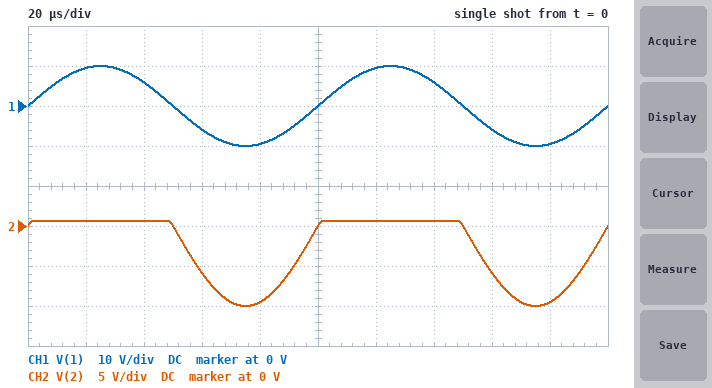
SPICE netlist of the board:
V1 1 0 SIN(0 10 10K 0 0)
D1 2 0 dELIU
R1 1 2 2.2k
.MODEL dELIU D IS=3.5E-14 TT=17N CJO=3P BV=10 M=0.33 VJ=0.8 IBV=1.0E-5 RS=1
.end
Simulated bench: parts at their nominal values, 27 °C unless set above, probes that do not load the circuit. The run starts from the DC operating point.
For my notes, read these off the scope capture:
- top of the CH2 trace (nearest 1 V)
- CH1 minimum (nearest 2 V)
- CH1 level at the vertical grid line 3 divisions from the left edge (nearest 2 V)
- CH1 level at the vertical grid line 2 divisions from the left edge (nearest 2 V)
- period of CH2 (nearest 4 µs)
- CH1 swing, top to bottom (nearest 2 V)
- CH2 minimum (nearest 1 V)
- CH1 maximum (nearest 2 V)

1 V
-10 V
-6 V
6 V
100 µs
20 V
-10 V
10 V
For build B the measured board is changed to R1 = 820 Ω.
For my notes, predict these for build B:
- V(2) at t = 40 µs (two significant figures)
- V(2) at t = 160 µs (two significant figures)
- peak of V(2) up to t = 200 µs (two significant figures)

680 mV
-5.9 V
700 mV
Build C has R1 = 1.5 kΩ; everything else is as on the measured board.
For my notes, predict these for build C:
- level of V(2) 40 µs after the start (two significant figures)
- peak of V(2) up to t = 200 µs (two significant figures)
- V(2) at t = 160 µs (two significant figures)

660 mV
680 mV
-5.9 V
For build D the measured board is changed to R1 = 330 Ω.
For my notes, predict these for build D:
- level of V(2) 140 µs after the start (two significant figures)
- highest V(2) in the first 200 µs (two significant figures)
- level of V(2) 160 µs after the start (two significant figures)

710 mV
740 mV
-5.9 V
